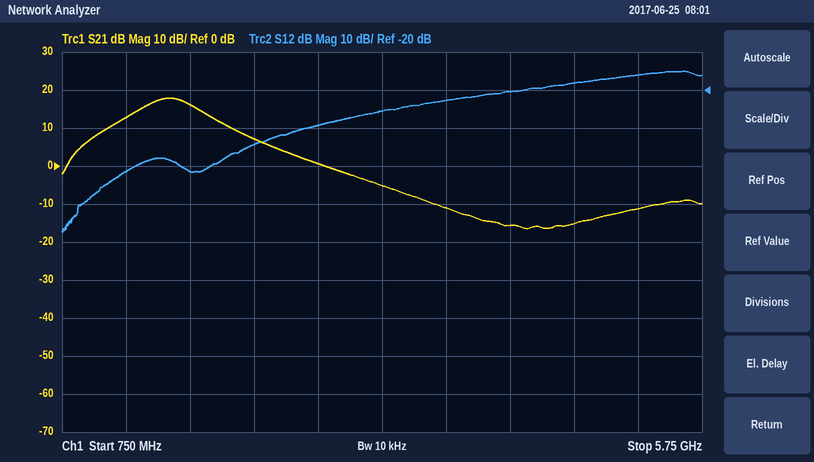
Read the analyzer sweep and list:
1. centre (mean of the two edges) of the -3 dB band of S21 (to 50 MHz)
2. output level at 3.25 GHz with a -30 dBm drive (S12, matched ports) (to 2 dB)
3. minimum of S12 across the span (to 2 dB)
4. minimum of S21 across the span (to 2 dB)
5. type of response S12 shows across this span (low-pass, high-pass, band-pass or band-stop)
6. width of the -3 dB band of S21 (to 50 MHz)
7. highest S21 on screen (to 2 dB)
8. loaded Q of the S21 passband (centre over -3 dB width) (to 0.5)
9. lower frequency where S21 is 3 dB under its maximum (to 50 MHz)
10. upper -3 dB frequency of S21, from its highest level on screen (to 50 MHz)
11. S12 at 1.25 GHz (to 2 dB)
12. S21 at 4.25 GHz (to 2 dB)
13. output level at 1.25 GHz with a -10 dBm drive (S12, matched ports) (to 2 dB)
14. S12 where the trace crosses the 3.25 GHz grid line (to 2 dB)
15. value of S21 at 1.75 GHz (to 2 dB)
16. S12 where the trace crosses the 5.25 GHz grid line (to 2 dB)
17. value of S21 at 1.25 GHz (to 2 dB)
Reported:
1.60 GHz
-56 dBm
-58 dB
-16 dB
high-pass
450 MHz
18 dB
3.5
1.35 GHz
1.80 GHz
-42 dB
-16 dB
-52 dBm
-26 dB
16 dB
-16 dB
12 dB
